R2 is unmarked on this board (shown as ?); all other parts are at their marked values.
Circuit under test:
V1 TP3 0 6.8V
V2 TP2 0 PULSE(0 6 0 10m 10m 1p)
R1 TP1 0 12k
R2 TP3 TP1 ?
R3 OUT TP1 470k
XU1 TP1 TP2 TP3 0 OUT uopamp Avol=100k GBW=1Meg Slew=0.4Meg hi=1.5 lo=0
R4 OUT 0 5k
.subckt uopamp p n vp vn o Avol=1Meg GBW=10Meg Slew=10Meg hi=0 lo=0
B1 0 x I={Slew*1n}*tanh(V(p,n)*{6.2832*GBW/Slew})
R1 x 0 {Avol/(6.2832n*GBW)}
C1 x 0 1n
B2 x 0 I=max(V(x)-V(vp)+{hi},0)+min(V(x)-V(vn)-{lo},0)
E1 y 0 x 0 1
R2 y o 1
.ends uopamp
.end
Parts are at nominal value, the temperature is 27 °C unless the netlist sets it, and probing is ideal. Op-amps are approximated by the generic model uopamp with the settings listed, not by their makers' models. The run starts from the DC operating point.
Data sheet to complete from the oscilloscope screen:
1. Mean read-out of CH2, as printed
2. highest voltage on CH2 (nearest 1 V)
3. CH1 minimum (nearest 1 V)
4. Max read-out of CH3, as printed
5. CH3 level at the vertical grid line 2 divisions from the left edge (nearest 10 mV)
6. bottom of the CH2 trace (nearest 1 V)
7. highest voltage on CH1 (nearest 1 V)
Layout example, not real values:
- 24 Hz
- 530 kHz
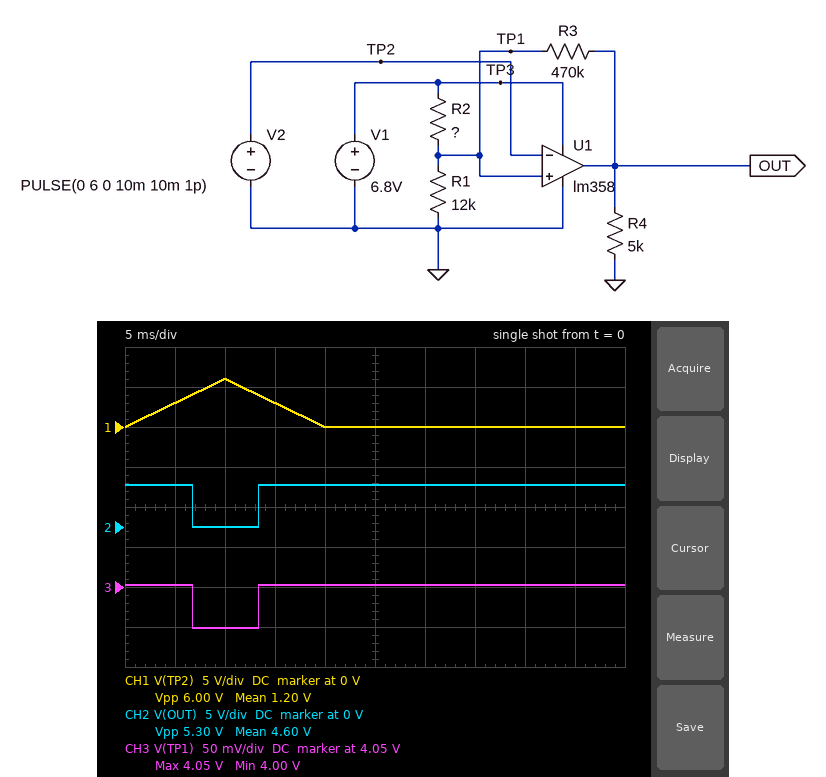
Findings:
- 4.60 V
- 5 V
- 0 V
- 4.05 V
- 4.00 V
- 0 V
- 6 V
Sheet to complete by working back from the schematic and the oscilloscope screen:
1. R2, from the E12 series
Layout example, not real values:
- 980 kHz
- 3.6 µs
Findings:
- 8.2 kΩ
